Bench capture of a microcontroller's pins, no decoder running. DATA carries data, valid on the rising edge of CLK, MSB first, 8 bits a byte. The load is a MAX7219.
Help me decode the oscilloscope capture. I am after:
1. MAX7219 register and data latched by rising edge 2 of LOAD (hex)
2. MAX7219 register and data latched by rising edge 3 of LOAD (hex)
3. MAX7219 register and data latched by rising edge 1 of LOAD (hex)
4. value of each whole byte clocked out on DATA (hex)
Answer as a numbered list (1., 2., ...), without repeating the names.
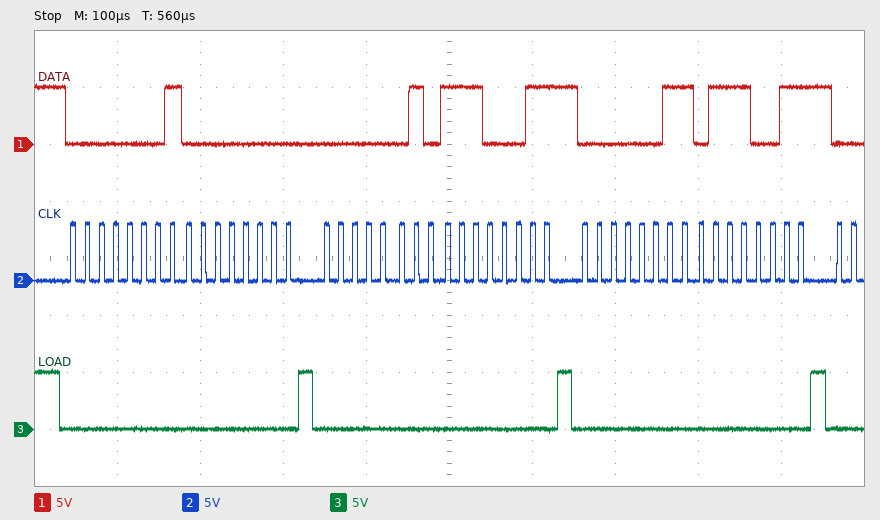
1. register 0x2, data 0xE3
2. register 0x3, data 0x73
3. register 0x1, data 0x00
4. 01 00 02 E3 03 73
